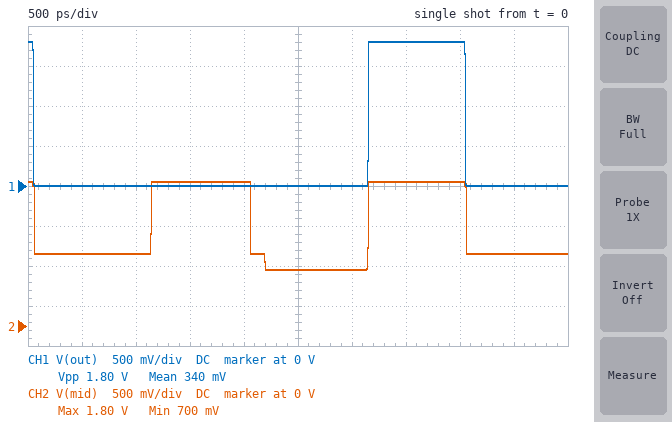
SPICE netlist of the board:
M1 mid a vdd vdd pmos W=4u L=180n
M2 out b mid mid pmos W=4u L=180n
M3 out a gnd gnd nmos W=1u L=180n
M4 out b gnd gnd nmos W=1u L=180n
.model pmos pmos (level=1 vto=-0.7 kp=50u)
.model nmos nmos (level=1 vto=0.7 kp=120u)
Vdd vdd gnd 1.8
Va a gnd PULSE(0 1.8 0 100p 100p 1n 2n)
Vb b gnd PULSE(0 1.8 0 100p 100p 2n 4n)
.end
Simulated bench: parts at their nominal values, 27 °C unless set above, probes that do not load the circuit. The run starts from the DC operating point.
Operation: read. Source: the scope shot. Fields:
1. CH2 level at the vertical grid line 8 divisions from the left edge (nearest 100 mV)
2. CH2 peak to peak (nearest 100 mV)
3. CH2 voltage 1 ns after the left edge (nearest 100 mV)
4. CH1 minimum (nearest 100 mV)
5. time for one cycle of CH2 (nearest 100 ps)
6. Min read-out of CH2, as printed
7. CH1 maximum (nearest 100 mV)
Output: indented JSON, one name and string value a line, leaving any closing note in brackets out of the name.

{
  "CH2 level at the vertical grid line 8 divisions from the left edge": "1.8 V",
  "CH2 peak to peak": "1.1 V",
  "CH2 voltage 1 ns after the left edge": "900 mV",
  "CH1 minimum": "0 V",
  "time for one cycle of CH2": "2.0 ns",
  "Min read-out of CH2, as printed": "700 mV",
  "CH1 maximum": "1.8 V"
}
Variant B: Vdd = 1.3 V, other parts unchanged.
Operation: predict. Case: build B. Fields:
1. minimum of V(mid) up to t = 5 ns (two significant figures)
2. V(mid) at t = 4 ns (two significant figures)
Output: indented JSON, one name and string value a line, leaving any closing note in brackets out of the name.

{
  "minimum of V(mid) up to t = 5 ns": "650 mV",
  "V(mid) at t = 4 ns": "1.3 V"
}
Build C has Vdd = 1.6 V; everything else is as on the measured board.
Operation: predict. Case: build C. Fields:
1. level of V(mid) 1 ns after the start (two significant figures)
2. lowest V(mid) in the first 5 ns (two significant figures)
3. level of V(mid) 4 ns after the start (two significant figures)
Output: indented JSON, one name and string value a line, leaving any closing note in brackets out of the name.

{
  "level of V(mid) 1 ns after the start": "800 mV",
  "lowest V(mid) in the first 5 ns": "700 mV",
  "level of V(mid) 4 ns after the start": "1.6 V"
}
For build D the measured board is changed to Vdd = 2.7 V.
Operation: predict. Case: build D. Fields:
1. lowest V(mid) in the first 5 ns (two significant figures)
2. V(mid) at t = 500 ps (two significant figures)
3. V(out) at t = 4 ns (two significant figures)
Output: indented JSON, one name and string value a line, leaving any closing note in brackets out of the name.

{
  "lowest V(mid) in the first 5 ns": "900 mV",
  "V(mid) at t = 500 ps": "2.6 V",
  "V(out) at t = 4 ns": "2.7 V"
}
